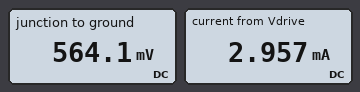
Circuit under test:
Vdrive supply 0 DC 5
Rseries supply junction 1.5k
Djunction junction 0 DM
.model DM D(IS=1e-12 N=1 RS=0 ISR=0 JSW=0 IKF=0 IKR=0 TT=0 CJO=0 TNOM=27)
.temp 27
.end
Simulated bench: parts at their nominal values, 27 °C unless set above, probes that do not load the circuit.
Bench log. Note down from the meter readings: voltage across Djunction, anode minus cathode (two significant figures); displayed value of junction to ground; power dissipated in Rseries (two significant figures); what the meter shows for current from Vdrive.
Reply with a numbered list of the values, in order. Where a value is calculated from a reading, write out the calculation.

1. 564.1 mV = 560 mV
2. 564.1 mV
3. (5 V - 564.1 mV)^2 / 1.5 kΩ = 13 mW
4. 2.957 mA
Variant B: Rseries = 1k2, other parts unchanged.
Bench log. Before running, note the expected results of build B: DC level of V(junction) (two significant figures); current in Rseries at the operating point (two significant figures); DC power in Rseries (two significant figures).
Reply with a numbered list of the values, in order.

1. 570 mV
2. 3.7 mA
3. 16 mW
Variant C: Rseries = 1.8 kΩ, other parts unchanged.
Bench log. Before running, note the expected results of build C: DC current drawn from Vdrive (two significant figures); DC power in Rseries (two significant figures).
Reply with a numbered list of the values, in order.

1. 2.5 mA
2. 11 mW
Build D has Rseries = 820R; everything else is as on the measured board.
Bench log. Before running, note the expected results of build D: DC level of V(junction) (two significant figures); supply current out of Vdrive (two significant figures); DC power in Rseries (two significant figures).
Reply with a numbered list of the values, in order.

1. 580 mV
2. 5.4 mA
3. 24 mW
